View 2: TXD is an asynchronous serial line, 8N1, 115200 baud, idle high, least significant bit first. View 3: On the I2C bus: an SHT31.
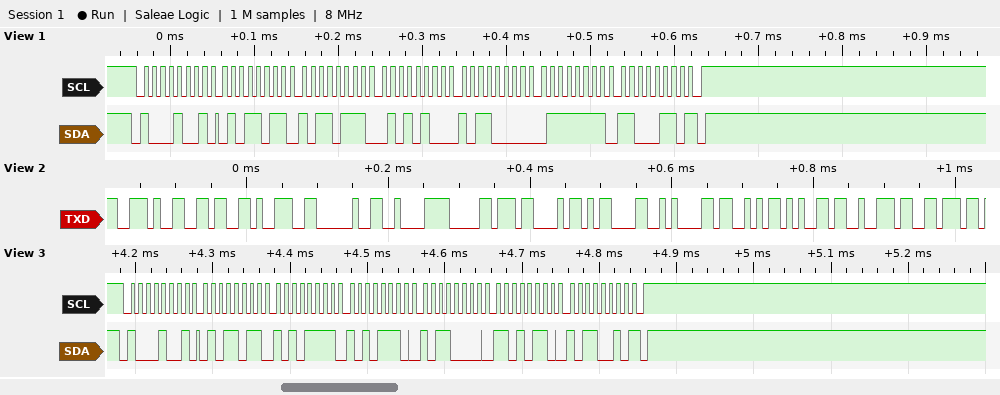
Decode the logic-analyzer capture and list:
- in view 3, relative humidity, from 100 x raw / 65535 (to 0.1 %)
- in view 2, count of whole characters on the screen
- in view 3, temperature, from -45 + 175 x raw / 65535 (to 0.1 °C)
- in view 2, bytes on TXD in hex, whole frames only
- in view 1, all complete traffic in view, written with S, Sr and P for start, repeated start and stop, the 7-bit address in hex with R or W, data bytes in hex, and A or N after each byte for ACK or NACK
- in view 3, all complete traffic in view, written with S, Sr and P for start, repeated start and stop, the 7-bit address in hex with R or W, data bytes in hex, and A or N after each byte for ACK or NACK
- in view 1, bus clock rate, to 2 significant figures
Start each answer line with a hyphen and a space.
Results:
- 69.1 %
- 13
- 17.7 °C
- 0x2E 0x36 0x39 0x20 0xC2 0xB0 0x43 0x0D 0x0A 0x53 0x65 0x72 0x76
- S 44R A 5B A B7 A 54 A B0 A 7F A C6 N P
- S 44R A 5B A AF A AE A B0 A D6 A B2 N P
- 100 kHz
